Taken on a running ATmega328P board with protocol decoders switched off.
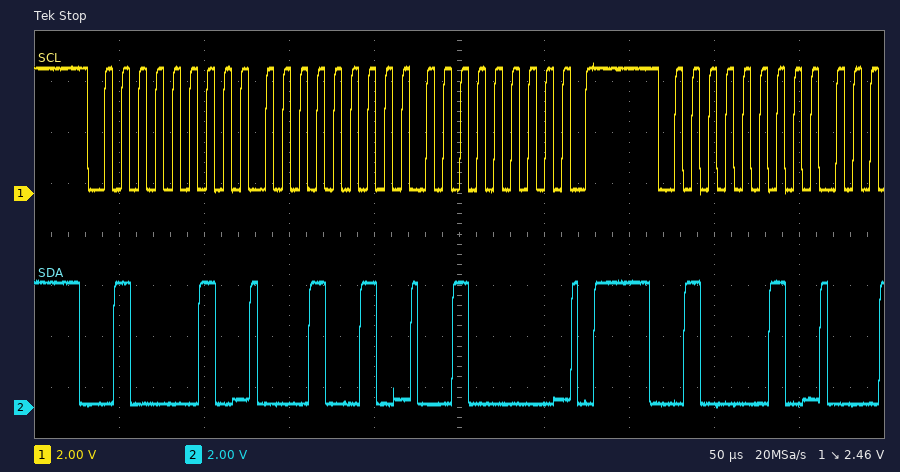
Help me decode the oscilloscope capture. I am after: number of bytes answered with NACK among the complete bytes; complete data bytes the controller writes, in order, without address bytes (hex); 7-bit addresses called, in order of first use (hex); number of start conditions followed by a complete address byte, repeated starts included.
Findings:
0
12 20
0x21
2
